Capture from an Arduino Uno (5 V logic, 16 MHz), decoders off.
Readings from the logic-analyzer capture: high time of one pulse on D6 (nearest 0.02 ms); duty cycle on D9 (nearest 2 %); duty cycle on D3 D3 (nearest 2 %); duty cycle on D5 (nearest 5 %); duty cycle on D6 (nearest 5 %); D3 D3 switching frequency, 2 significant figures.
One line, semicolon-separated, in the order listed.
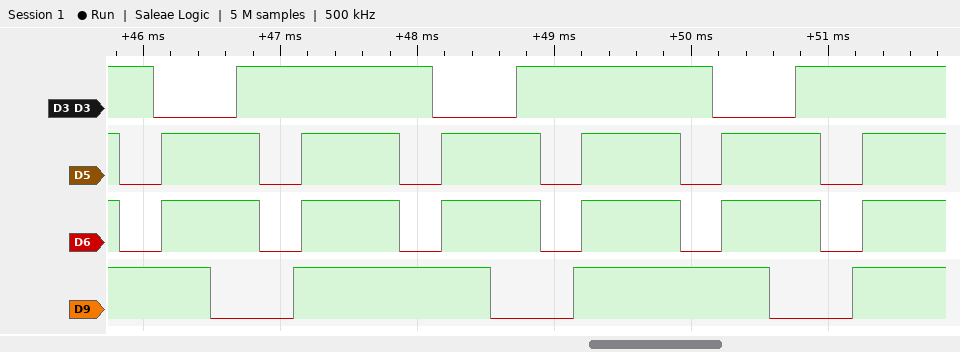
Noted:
0.72 ms; 70 %; 70 %; 70 %; 70 %; 490 Hz
